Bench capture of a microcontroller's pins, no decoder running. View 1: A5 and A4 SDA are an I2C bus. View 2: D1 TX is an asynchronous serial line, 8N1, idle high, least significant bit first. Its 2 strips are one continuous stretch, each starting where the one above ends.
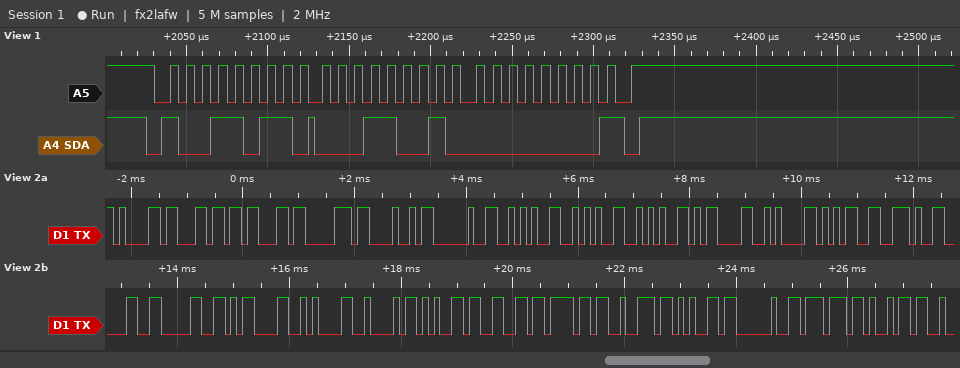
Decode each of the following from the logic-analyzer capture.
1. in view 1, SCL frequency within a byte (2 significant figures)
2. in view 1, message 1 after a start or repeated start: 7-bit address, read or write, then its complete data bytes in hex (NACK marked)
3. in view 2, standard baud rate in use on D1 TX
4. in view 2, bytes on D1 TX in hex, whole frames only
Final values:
100 kHz
0x4D read: 19 00 NACK
9600 baud
61 6C 63 70 48 20 2A 2A 2A 0D 0A 35 2E 30 30 0D 0A 42 65 66 6F 72 65 20 77 69
